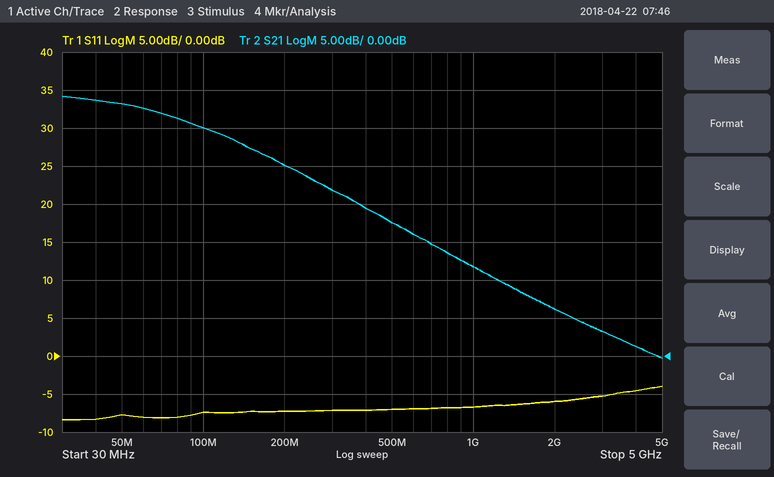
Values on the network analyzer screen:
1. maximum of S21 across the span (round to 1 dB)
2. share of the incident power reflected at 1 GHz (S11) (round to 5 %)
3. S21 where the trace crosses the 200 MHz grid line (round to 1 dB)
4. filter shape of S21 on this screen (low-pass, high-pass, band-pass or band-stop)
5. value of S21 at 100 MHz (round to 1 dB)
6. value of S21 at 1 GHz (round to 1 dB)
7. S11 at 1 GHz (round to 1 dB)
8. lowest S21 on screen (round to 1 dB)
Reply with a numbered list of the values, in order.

1. 34 dB
2. 20 %
3. 25 dB
4. low-pass
5. 30 dB
6. 12 dB
7. -7 dB
8. 0 dB
